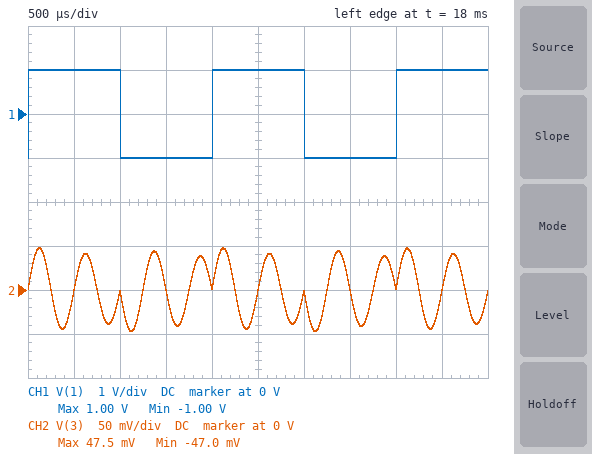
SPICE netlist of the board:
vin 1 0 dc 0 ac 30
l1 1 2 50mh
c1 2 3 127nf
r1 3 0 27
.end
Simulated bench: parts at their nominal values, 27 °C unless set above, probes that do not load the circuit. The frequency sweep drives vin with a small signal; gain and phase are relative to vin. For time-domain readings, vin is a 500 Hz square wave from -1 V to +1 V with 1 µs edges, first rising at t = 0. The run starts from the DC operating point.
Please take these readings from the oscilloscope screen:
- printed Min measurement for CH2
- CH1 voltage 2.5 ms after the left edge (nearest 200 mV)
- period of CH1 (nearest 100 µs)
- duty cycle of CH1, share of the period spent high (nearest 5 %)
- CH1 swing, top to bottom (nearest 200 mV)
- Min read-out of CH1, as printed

-47.0 mV
1.0 V
2.0 ms
50 %
2.0 V
-1.00 V
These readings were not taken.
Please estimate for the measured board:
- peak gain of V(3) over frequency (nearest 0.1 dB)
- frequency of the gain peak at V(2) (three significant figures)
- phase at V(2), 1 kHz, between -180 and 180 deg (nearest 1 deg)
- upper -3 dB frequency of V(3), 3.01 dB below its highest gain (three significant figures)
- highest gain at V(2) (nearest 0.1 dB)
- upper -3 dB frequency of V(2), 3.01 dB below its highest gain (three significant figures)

0 dB
2.00 kHz
0 deg
2.04 kHz
27.3 dB
2.04 kHz
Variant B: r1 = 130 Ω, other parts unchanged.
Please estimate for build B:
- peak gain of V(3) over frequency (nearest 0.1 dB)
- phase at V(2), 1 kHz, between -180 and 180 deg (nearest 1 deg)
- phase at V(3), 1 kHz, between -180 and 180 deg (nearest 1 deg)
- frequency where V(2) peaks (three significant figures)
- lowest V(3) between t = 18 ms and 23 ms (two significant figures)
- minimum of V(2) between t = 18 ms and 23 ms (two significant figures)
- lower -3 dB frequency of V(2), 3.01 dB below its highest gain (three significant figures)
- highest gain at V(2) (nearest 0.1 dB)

0 dB
-2 deg
82 deg
1.98 kHz
-280 mV
-2.2 V
1.76 kHz
13.9 dB
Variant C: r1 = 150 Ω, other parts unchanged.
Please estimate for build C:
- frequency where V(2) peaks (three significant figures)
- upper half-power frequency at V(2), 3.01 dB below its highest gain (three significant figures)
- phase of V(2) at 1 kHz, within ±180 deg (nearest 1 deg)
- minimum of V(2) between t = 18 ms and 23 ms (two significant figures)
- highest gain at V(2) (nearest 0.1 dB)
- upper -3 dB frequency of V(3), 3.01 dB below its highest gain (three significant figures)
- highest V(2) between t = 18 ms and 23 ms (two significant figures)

1.97 kHz
2.20 kHz
-2 deg
-2.2 V
12.7 dB
2.25 kHz
2.2 V
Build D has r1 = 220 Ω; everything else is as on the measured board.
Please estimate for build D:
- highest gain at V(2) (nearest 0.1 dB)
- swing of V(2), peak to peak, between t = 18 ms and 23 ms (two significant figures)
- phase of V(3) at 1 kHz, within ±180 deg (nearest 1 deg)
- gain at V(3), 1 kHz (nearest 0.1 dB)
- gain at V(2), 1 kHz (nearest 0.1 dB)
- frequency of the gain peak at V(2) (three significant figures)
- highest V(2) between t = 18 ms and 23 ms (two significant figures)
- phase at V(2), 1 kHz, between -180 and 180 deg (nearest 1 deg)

9.7 dB
4.2 V
77 deg
-12.8 dB
2.4 dB
1.94 kHz
2.1 V
-3 deg
